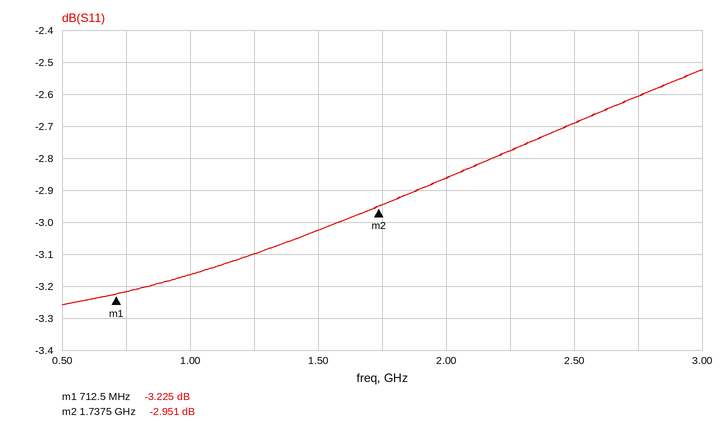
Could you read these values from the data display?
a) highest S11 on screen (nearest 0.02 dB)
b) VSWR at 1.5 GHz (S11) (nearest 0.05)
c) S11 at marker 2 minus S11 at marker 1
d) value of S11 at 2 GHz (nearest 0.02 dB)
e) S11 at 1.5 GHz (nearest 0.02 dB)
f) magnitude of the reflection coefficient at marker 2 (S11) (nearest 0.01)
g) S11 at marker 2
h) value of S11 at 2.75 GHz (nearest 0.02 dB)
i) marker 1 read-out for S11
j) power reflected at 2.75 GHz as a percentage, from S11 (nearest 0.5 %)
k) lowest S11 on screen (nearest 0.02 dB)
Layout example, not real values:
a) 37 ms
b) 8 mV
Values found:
a) -2.52 dB
b) 5.80
c) 0.274 dB
d) -2.86 dB
e) -3.02 dB
f) 0.71
g) -2.951 dB
h) -2.60 dB
i) -3.225 dB
j) 55.0 %
k) -3.26 dB
